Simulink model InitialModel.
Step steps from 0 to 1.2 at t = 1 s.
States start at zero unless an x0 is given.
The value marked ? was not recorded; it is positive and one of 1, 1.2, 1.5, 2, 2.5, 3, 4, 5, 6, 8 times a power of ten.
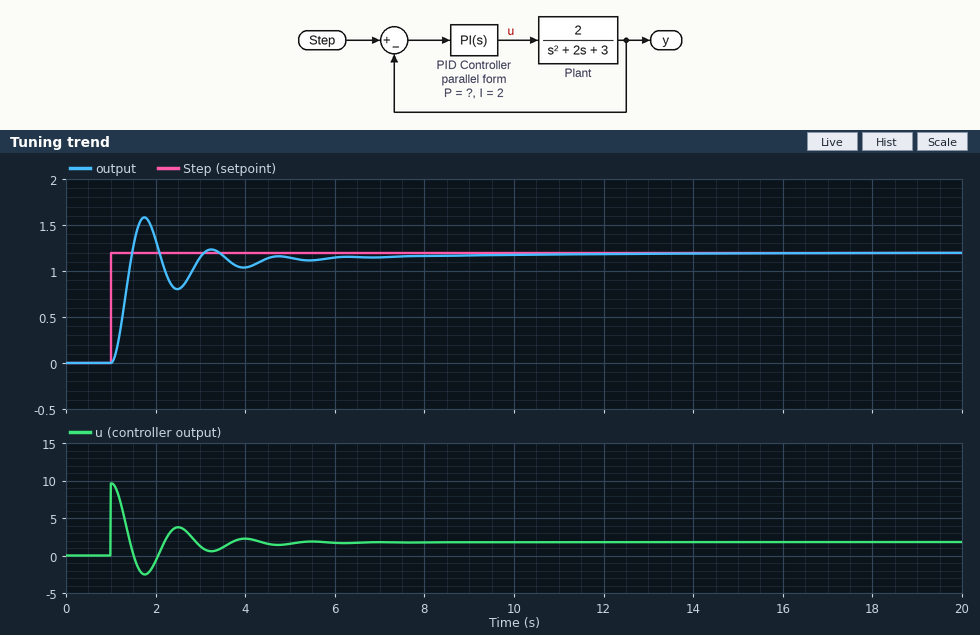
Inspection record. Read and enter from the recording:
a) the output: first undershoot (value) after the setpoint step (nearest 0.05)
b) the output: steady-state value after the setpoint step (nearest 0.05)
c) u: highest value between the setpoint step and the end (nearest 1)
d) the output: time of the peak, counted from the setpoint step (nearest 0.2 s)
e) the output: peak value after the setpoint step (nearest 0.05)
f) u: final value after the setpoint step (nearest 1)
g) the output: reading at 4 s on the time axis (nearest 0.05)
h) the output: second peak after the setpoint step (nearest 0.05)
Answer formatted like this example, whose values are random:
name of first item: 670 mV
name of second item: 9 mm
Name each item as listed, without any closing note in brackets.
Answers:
the output: first undershoot (value) after the setpoint step: 0.80
the output: steady-state value after the setpoint step: 1.20
u: highest value between the setpoint step and the end: 10
the output: time of the peak, counted from the setpoint step: 0.8 s
the output: peak value after the setpoint step: 1.60
u: final value after the setpoint step: 2
the output: reading at 4 s on the time axis: 1.05
the output: second peak after the setpoint step: 1.25
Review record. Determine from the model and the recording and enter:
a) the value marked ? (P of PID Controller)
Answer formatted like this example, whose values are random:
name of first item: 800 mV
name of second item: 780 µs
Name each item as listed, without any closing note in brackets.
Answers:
the value marked ?: 8
